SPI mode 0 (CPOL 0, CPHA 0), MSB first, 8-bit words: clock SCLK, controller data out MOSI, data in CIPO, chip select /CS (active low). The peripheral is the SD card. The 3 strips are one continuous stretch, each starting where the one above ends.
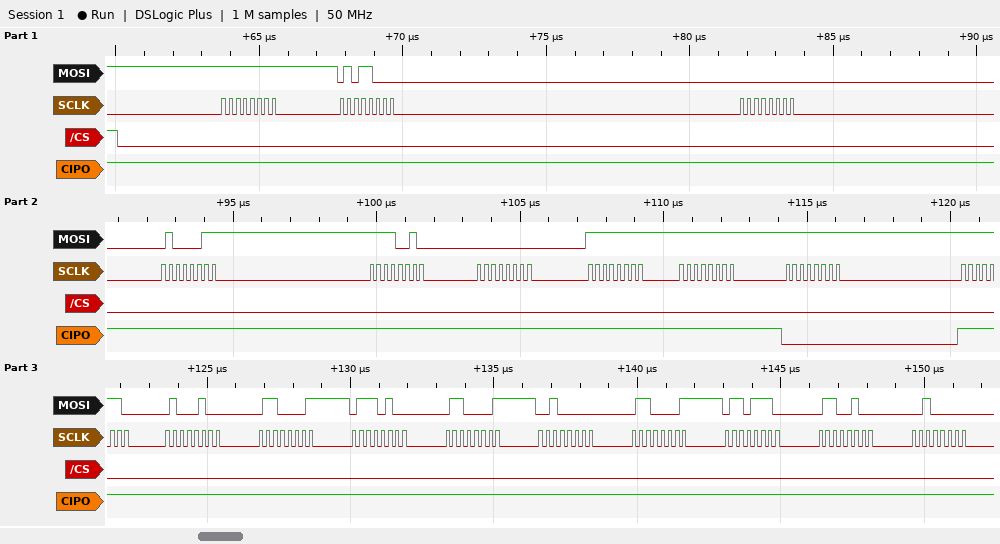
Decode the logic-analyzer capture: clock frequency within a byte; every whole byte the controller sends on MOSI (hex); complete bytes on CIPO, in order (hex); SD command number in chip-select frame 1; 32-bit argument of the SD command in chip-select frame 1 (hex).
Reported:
4 MHz
FF 58 00 43 F2 00 FF FF FF FE 44 61 74 61 20 61 6E 64 20
FF FF FF FF FF FF FF FF 00 FF FF FF FF FF FF FF FF FF FF
CMD24
0x0043F200
